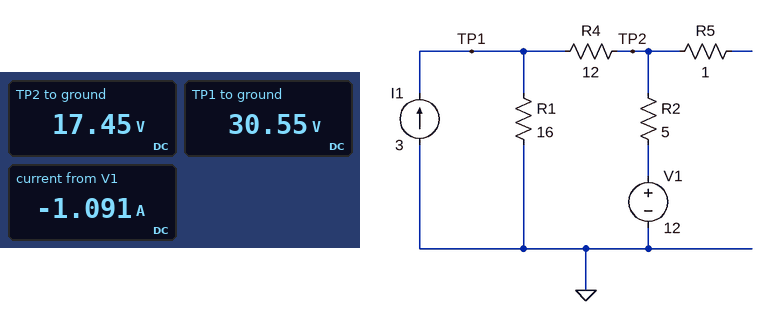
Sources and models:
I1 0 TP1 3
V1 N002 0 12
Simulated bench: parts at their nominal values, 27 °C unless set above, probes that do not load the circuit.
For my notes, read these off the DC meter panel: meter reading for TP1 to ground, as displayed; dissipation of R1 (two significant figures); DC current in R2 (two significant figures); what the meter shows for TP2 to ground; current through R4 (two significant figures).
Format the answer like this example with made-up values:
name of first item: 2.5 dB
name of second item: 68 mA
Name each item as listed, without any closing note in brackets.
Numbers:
meter reading for TP1 to ground, as displayed: 30.55 V
dissipation of R1: 58 W
DC current in R2: 1.1 A
what the meter shows for TP2 to ground: 17.45 V
current through R4: 1.1 A
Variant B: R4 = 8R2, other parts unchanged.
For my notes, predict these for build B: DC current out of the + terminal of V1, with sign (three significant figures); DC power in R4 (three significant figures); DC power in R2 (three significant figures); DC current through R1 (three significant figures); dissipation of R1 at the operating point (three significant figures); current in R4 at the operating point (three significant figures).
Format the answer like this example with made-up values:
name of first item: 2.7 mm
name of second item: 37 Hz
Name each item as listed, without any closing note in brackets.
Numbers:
DC current out of the + terminal of V1, with sign: -1.23 A
DC power in R4: 12.5 W
DC power in R2: 7.60 W
DC current through R1: 1.77 A
dissipation of R1 at the operating point: 50.0 W
current in R4 at the operating point: 1.23 A
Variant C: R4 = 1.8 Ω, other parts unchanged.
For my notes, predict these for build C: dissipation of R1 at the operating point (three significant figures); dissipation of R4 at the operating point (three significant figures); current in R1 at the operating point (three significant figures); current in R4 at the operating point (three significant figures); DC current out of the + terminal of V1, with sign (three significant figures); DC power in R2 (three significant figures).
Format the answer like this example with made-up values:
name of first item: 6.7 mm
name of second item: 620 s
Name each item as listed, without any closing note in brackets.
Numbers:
dissipation of R1 at the operating point: 32.3 W
dissipation of R4 at the operating point: 4.49 W
current in R1 at the operating point: 1.42 A
current in R4 at the operating point: 1.58 A
DC current out of the + terminal of V1, with sign: -1.58 A
DC power in R2: 12.5 W
